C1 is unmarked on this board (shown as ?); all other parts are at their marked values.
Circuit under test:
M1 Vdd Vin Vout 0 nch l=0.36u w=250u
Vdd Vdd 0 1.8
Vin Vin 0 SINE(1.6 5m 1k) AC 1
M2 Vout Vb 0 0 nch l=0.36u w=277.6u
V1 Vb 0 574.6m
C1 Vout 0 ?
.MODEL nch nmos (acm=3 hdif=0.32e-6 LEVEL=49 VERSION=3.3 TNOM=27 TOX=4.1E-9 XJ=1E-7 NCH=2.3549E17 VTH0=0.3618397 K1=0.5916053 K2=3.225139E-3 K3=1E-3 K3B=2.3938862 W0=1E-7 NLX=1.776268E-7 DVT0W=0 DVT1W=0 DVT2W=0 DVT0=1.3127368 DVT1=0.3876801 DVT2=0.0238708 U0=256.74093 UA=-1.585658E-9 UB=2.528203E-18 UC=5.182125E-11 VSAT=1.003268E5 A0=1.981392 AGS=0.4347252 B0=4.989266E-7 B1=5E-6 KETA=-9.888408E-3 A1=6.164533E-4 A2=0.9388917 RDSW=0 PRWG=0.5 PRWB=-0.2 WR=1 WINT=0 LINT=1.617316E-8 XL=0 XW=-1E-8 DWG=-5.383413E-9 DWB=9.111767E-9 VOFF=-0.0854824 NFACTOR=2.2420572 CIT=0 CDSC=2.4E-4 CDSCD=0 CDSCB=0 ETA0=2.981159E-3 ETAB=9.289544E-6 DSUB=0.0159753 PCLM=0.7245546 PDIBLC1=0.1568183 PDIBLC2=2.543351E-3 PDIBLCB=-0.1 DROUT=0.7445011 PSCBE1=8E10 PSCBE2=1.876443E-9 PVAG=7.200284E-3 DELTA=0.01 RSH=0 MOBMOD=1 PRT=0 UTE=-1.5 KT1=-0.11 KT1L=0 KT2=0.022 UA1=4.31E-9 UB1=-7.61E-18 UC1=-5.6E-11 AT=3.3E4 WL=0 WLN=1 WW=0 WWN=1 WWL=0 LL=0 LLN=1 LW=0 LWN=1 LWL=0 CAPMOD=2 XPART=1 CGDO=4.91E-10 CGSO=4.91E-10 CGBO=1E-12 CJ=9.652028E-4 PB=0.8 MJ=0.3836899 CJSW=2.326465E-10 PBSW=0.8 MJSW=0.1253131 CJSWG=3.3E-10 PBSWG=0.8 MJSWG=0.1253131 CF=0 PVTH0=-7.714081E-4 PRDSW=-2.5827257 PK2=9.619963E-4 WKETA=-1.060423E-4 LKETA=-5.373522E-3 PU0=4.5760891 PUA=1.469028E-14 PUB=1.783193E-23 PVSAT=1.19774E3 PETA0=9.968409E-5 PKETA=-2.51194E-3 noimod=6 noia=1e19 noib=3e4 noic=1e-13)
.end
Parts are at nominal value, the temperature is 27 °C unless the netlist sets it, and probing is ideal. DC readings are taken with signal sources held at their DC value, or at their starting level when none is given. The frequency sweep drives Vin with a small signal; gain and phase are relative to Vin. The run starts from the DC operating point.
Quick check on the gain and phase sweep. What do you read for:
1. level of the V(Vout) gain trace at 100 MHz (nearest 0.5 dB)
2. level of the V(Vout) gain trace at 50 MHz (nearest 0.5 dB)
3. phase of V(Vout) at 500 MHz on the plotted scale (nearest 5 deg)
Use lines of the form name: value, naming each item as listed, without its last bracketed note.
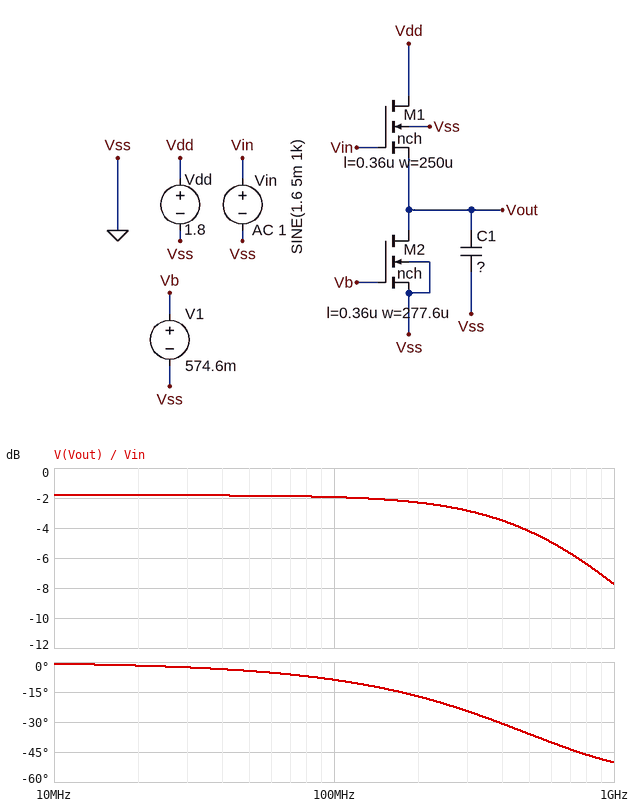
level of the V(Vout) gain trace at 100 MHz: -2.0 dB
level of the V(Vout) gain trace at 50 MHz: -2.0 dB
phase of V(Vout) at 500 MHz on the plotted scale: -35 deg
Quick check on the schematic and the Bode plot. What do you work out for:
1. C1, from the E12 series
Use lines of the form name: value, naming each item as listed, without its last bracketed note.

C1, from the E12 series: 5.6 pF
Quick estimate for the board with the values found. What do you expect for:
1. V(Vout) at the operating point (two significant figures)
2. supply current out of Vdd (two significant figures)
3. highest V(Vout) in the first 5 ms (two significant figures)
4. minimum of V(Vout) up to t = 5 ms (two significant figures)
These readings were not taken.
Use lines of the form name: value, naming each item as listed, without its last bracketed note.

V(Vout) at the operating point: 830 mV
supply current out of Vdd: 1.3 mA
highest V(Vout) in the first 5 ms: 830 mV
minimum of V(Vout) up to t = 5 ms: 820 mV
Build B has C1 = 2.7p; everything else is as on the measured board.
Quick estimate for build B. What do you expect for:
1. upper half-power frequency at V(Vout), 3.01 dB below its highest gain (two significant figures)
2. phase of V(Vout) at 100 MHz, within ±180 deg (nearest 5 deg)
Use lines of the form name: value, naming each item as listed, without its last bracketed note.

upper half-power frequency at V(Vout), 3.01 dB below its highest gain: 1.0 GHz
phase of V(Vout) at 100 MHz, within ±180 deg: -5 deg
